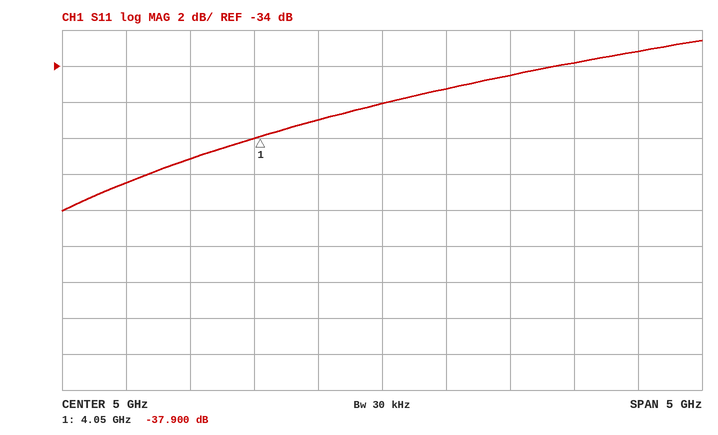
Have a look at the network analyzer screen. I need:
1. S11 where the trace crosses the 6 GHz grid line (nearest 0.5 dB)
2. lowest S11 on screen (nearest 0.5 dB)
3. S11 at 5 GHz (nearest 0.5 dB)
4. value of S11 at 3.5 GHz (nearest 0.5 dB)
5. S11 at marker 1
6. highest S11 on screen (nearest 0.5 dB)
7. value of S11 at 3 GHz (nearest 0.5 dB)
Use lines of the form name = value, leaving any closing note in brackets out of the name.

S11 where the trace crosses the 6 GHz grid line = -34.5 dB
lowest S11 on screen = -42.0 dB
S11 at 5 GHz = -36.0 dB
value of S11 at 3.5 GHz = -39.0 dB
S11 at marker 1 = -37.900 dB
highest S11 on screen = -32.5 dB
value of S11 at 3 GHz = -40.5 dB
